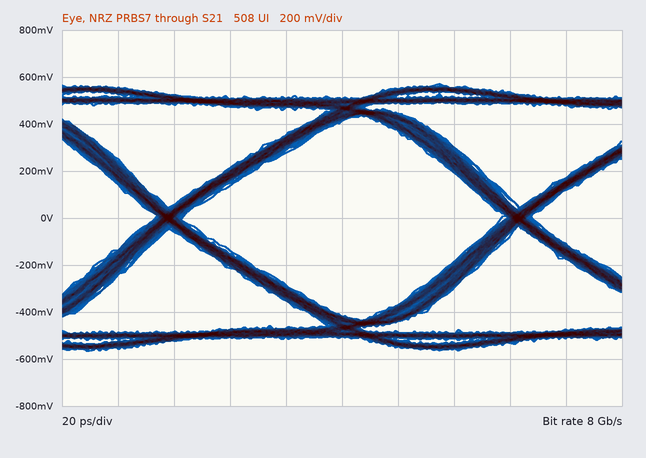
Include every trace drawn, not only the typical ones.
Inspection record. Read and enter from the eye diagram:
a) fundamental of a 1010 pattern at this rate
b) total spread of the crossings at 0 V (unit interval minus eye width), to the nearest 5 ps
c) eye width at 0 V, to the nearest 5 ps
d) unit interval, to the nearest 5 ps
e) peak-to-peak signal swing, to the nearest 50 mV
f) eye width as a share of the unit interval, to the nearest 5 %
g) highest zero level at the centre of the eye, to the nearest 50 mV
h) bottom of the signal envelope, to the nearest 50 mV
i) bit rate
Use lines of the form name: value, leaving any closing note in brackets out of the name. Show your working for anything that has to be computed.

fundamental of a 1010 pattern at this rate: 4 GHz
total spread of the crossings at 0 V (unit interval minus eye width), to the nearest 5 ps: 10 ps
eye width at 0 V, to the nearest 5 ps: 115 ps
unit interval, to the nearest 5 ps: 125 ps
peak-to-peak signal swing, to the nearest 50 mV: 1.15 V
eye width as a share of the unit interval, to the nearest 5 %: 115 ps / 125 ps ≈ 92.0 %, so 90 % to the nearest 5 %
highest zero level at the centre of the eye, to the nearest 50 mV: -400 mV
bottom of the signal envelope, to the nearest 50 mV: -550 mV
bit rate: 8 Gb/s
